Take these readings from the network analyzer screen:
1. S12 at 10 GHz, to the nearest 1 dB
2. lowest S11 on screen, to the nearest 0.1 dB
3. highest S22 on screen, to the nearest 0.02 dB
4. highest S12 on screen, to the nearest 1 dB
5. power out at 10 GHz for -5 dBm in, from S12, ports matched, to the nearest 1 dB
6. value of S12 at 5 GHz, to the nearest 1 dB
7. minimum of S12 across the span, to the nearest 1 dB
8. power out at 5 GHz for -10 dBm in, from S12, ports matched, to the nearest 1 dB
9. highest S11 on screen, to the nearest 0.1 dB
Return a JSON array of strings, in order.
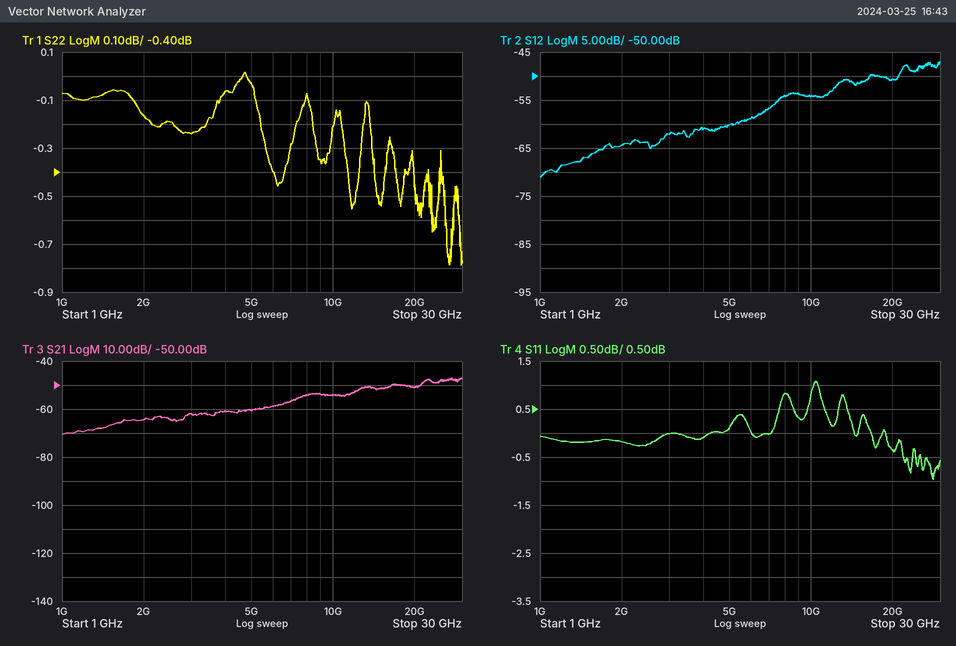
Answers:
["-54 dB", "-1.0 dB", "0.02 dB", "-47 dB", "-59 dBm", "-60 dB", "-71 dB", "-70 dBm", "1.1 dB"]
